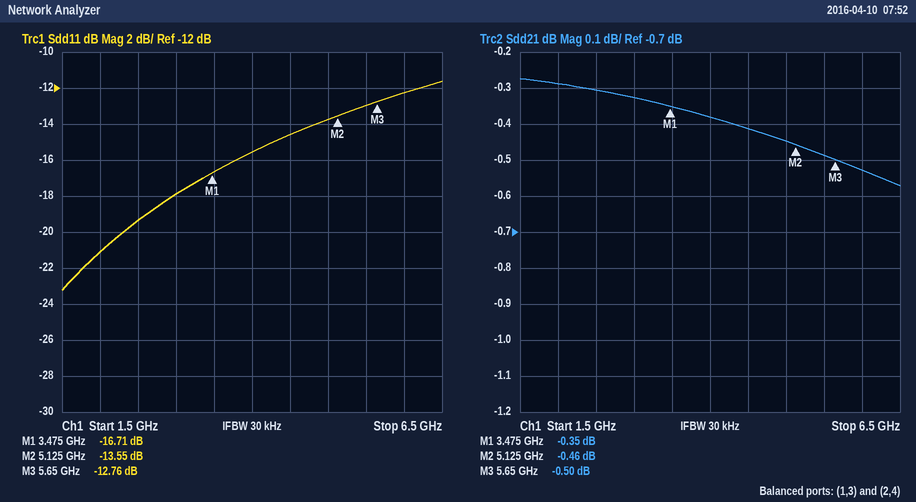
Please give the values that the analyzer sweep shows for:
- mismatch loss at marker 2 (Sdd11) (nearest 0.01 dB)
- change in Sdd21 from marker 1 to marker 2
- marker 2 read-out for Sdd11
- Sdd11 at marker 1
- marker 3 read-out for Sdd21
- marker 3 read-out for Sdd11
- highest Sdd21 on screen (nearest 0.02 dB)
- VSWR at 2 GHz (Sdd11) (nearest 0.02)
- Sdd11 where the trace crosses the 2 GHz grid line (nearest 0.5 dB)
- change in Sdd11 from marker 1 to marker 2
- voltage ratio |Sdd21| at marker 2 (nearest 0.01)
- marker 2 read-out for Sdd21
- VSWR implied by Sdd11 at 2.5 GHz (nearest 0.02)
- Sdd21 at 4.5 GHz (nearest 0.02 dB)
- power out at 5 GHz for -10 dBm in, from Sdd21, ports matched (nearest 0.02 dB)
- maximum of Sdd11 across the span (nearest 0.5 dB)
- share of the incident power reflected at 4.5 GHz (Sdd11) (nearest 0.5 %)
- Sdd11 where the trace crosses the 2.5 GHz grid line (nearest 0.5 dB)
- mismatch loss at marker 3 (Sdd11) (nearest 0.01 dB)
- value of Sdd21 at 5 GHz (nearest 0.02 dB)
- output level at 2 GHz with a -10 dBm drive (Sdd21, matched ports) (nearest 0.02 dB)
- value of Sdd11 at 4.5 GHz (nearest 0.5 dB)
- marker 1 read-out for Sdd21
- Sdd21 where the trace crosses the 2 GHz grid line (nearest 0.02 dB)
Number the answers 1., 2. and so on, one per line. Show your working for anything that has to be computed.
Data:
1. −10 log10(1 − 10^(-13.55/10)) ≈ 0.20 dB
2. -0.46 − (-0.35) = -0.11 dB
3. -13.55 dB
4. -16.71 dB
5. -0.50 dB
6. -12.76 dB
7. -0.28 dB
8. |Γ| = 10^(-21/20) = 0.0891; VSWR = (1 + 0.0891)/(1 − 0.0891) ≈ 1.20
9. -21.0 dB
10. -13.55 − (-16.71) = 3.16 dB
11. 10^(-0.46/20) ≈ 0.95
12. -0.46 dB
13. |Γ| = 10^(-19.5/20) = 0.1059; VSWR = (1 + 0.1059)/(1 − 0.1059) ≈ 1.24
14. -0.42 dB
15. -10 dBm + (-0.44 dB) = -10.44 dBm
16. -11.5 dB
17. 10^(-14.5/10) ≈ 3.5 %
18. -19.5 dB
19. −10 log10(1 − 10^(-12.76/10)) ≈ 0.24 dB
20. -0.44 dB
21. -10 dBm + (-0.28 dB) = -10.28 dBm
22. -14.5 dB
23. -0.35 dB
24. -0.28 dB
